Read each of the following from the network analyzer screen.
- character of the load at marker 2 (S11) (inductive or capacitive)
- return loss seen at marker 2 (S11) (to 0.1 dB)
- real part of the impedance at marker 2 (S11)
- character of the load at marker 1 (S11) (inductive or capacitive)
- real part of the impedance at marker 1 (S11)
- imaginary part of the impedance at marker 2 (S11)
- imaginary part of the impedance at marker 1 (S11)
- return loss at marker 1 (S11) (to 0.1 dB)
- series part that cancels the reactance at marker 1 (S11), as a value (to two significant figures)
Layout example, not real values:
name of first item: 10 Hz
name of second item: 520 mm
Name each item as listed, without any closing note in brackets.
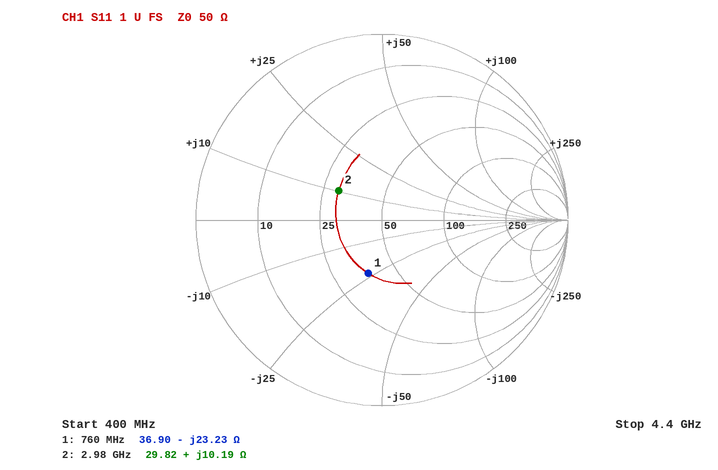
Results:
character of the load at marker 2 (S11): inductive
return loss seen at marker 2 (S11): 11.0 dB
real part of the impedance at marker 2: 29.82 Ω
character of the load at marker 1 (S11): capacitive
real part of the impedance at marker 1: 36.90 Ω
imaginary part of the impedance at marker 2: +10.19 Ω
imaginary part of the impedance at marker 1: -23.23 Ω
return loss at marker 1 (S11): 10.6 dB
series part that cancels the reactance at marker 1 (S11), as a value: 4.9 nH
